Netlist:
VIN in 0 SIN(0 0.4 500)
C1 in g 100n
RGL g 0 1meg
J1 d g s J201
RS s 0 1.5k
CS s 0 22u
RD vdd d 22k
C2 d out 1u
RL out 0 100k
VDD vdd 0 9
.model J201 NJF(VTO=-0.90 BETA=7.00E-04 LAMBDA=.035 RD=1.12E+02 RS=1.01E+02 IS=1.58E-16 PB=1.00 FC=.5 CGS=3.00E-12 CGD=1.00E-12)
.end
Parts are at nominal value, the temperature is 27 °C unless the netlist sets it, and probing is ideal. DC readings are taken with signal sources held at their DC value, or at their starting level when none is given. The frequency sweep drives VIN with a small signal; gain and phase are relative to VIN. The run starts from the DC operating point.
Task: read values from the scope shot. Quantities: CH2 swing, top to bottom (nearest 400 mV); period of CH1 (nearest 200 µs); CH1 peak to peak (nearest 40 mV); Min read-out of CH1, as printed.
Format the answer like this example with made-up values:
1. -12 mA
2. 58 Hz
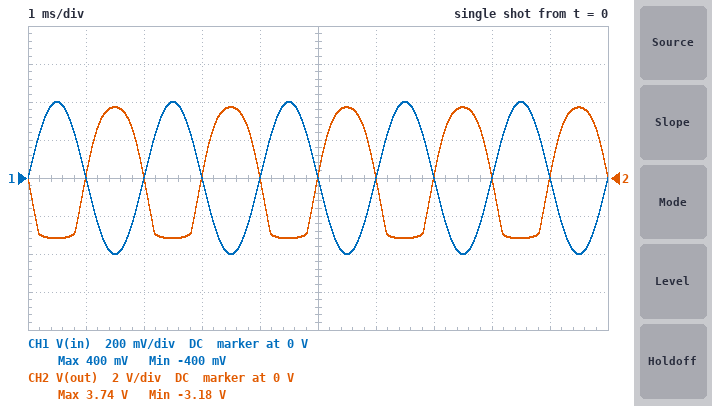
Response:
1. 6.8 V
2. 2.0 ms
3. 800 mV
4. -400 mV
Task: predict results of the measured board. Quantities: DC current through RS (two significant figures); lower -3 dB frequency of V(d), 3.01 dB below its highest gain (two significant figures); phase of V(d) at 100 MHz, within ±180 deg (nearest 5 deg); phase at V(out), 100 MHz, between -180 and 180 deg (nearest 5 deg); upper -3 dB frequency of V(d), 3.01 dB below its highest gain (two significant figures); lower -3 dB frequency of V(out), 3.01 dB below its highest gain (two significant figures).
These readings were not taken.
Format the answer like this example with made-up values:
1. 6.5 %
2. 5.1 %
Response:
1. 230 µA
2. 7.5 Hz
3. 75 deg
4. 75 deg
5. 22 MHz
6. 7.9 Hz
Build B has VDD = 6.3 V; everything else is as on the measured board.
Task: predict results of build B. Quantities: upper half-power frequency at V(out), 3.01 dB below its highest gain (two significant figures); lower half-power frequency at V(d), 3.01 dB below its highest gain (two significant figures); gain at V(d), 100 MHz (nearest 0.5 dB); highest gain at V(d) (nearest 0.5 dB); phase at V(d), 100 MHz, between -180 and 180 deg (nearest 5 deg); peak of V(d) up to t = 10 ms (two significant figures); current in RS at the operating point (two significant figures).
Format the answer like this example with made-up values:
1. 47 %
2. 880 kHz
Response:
1. 16 MHz
2. 7.2 Hz
3. 6.5 dB
4. 21.5 dB
5. 65 deg
6. 5.0 V
7. 220 µA
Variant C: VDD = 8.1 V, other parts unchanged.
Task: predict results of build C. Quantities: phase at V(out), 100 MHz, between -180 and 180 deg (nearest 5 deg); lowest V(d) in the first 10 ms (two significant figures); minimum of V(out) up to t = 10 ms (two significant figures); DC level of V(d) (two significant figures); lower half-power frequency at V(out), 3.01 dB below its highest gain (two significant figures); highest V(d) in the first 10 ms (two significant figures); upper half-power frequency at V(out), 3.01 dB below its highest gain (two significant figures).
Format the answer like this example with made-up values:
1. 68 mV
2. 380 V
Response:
1. 70 deg
2. 740 mV
3. -2.4 V
4. 3.2 V
5. 7.8 Hz
6. 6.8 V
7. 20 MHz
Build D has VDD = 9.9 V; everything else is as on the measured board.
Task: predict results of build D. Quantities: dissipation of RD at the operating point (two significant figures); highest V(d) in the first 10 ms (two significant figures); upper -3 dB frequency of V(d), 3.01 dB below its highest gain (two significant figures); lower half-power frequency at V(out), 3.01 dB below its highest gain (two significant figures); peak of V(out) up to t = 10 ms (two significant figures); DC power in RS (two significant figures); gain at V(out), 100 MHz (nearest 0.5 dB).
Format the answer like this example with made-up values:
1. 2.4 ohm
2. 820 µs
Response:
1. 1.2 mW
2. 8.6 V
3. 24 MHz
4. 8.1 Hz
5. 3.8 V
6. 79 µW
7. 10.0 dB
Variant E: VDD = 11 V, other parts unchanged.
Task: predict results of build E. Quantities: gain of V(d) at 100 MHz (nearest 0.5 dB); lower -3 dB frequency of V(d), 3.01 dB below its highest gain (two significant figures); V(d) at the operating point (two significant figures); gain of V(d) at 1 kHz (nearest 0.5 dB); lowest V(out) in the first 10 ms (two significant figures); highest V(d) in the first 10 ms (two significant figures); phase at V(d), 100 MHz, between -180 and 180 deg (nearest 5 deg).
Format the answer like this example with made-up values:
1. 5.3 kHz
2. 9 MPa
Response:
1. 11.0 dB
2. 7.8 Hz
3. 5.9 V
4. 22.5 dB
5. -4.8 V
6. 9.7 V
7. 80 deg
